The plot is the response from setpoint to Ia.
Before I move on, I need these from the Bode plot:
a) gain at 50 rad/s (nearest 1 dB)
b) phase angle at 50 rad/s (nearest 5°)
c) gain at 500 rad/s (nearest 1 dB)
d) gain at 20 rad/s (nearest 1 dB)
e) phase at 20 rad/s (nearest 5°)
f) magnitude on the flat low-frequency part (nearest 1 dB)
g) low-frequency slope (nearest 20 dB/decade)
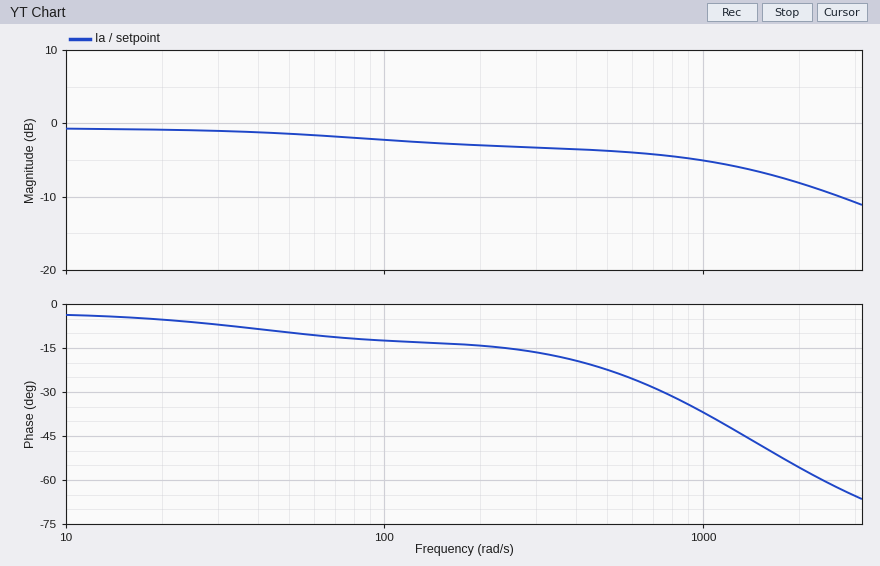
-1 dB
-10°
-4 dB
-1 dB
-5°
-1 dB
0 dB/decade
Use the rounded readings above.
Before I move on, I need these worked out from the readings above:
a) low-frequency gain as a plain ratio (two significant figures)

0.89
